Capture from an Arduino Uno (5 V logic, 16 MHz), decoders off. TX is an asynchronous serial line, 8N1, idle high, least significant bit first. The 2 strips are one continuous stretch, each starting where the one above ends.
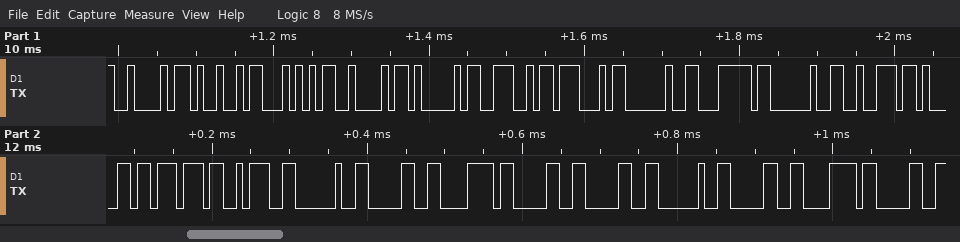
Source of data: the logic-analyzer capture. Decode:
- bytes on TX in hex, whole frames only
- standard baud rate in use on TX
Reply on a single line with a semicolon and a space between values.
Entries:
42 49 54 42 41 4E 47 20 7C 20 72 61 77 3A 20 30 78 30 30 20 30 78 30; 115200 baud
